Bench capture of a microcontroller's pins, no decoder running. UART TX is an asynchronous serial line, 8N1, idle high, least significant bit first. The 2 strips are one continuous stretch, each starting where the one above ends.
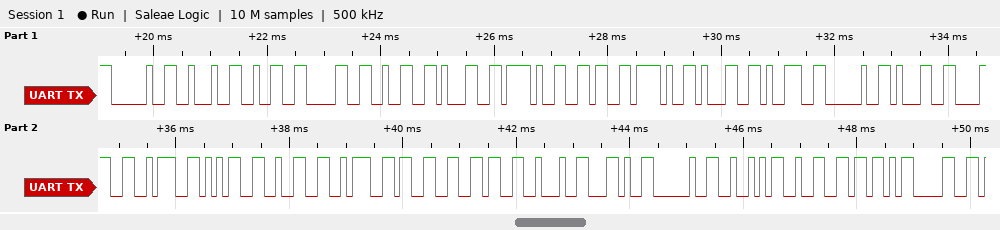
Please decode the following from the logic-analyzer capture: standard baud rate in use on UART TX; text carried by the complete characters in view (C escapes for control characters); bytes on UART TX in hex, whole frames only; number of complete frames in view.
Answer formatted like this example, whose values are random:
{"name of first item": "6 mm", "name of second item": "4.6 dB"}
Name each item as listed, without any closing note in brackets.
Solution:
{"standard baud rate in use on UART TX": "9600 baud", "text carried by the complete characters in view": "\" \\\"2021/6/19 18:52:36\\\", R2[0\"", "bytes on UART TX in hex, whole frames only": "0x20 0x22 0x32 0x30 0x32 0x31 0x2F 0x36 0x2F 0x31 0x39 0x20 0x31 0x38 0x3A 0x35 0x32 0x3A 0x33 0x36 0x22 0x2C 0x20 0x52 0x32 0x5B 0x30", "number of complete frames in view": "27"}
